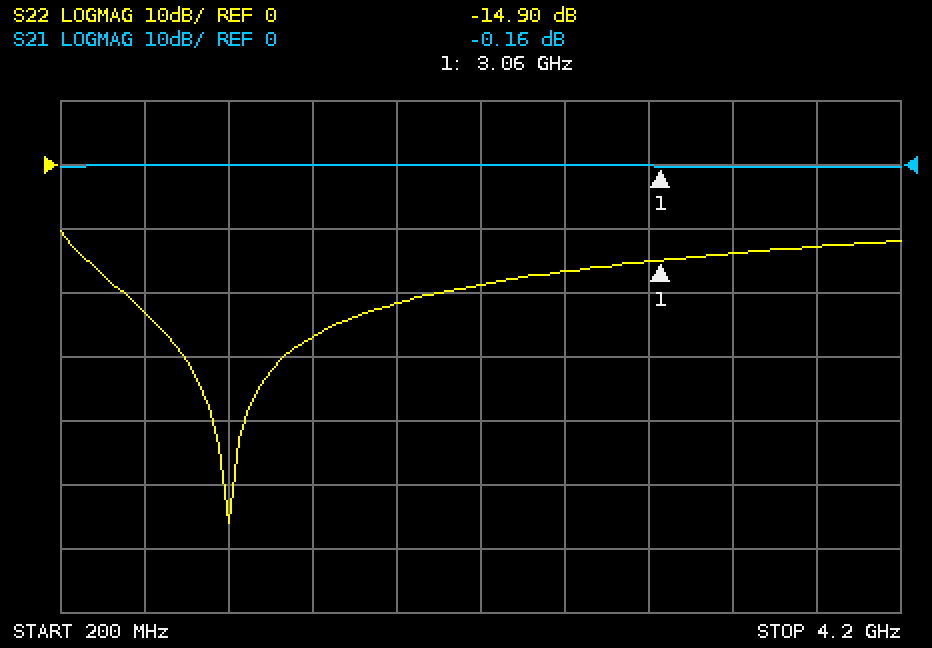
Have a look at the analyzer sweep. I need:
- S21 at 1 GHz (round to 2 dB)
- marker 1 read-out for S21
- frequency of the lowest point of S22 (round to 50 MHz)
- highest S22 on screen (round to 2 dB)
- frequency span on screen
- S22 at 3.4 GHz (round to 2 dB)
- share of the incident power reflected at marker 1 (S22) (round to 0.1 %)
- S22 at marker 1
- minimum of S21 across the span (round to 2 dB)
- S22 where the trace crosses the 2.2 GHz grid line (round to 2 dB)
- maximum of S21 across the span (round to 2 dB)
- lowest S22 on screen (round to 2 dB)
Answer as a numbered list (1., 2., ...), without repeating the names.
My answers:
1. 0 dB
2. -0.16 dB
3. 1.00 GHz
4. -10 dB
5. 4 GHz
6. -14 dB
7. 3.2 %
8. -14.90 dB
9. 0 dB
10. -18 dB
11. 0 dB
12. -56 dB
